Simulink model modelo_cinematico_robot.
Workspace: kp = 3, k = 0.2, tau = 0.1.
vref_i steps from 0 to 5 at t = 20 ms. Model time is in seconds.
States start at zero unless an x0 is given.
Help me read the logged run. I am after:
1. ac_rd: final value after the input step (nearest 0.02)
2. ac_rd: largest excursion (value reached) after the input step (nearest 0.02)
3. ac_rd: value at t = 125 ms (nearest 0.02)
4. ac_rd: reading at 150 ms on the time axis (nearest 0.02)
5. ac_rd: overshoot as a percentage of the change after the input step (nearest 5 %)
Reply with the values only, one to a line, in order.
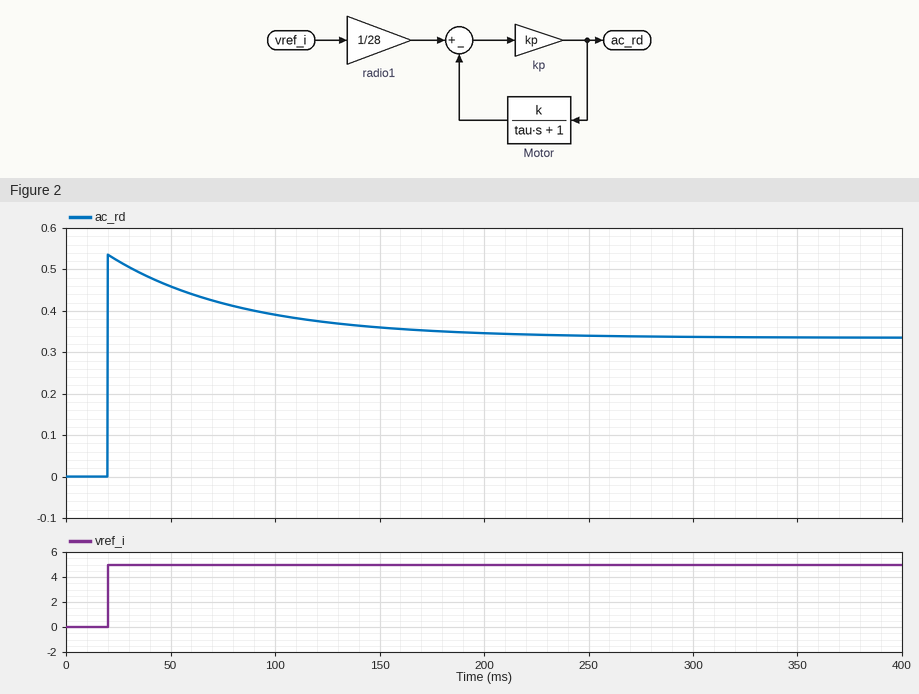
0.34
0.54
0.38
0.36
60 %
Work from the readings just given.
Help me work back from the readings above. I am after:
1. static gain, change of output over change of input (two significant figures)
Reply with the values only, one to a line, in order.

0.068
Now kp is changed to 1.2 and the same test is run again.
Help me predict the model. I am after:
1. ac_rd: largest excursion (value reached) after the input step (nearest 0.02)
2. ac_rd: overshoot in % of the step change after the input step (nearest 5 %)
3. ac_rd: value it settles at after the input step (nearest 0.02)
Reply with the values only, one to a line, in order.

0.22
25 %
0.18
